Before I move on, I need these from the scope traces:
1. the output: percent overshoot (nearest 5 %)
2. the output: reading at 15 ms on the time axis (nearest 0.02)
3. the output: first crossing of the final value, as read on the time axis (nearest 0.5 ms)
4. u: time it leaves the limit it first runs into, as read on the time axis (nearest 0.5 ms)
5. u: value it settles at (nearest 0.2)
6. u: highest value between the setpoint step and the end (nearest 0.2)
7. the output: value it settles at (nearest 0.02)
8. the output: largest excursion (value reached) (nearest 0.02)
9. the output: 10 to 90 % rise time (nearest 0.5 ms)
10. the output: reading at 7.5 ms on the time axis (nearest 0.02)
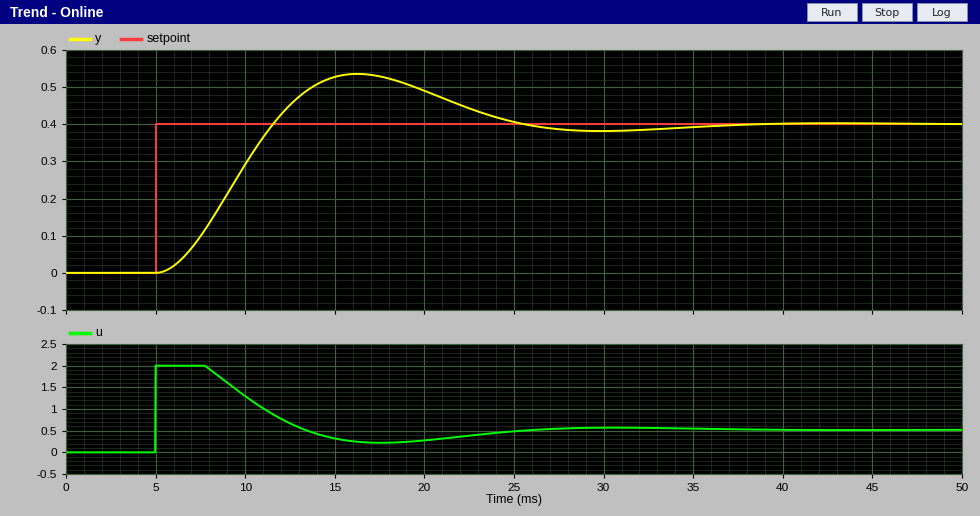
35 %
0.52
11.5 ms
8.0 ms
0.6
2.0
0.40
0.54
4.5 ms
0.10
